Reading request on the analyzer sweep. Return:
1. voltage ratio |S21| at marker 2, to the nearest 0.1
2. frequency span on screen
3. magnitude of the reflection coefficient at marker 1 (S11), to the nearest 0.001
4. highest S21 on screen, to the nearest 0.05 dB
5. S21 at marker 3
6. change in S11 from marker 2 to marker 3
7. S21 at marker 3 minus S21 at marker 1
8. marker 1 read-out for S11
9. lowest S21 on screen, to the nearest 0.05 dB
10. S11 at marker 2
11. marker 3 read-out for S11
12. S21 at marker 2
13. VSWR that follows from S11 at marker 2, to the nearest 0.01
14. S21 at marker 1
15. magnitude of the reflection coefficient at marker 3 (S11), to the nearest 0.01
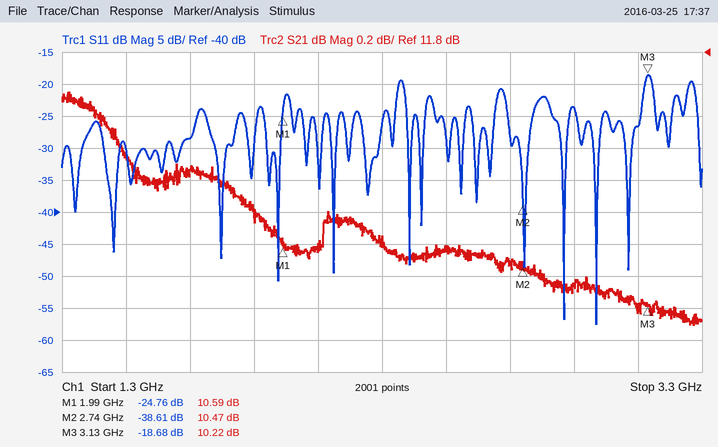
3.3
2 GHz
0.058
11.55 dB
10.22 dB
19.93 dB
-0.37 dB
-24.76 dB
10.10 dB
-38.61 dB
-18.68 dB
10.47 dB
1.02
10.59 dB
0.12
